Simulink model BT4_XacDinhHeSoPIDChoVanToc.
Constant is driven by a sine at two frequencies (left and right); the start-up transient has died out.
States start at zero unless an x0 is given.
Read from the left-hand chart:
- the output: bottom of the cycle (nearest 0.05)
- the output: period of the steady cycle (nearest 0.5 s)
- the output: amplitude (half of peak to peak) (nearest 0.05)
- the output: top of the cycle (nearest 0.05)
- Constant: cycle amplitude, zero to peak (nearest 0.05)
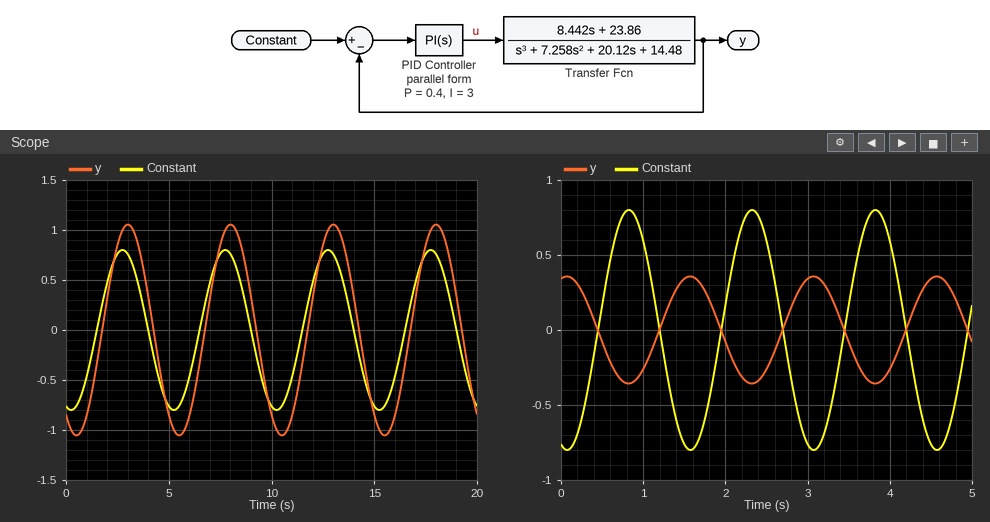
-1.05
5.0 s
1.05
1.05
0.80
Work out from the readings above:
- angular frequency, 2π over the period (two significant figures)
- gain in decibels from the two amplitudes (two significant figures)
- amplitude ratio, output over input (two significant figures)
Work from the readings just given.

1.3 rad/s
2.4 dB
1.3
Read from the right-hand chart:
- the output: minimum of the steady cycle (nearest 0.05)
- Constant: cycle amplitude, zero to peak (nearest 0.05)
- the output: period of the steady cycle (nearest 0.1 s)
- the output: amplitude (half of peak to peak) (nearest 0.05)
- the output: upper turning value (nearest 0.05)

-0.35
0.80
1.5 s
0.35
0.35
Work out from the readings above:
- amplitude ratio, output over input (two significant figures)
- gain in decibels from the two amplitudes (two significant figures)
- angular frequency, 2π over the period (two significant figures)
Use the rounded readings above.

0.44
-7.2 dB
4.2 rad/s
